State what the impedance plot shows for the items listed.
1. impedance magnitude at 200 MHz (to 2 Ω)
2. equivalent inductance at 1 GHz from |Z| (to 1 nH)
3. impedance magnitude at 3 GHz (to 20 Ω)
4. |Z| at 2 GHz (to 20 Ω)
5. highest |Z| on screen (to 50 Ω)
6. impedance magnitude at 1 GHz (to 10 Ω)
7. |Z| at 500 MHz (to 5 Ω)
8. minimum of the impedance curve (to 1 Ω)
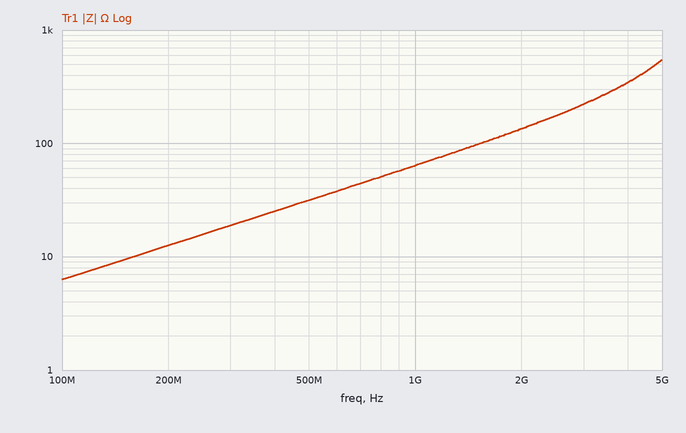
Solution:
12 Ω
10 nH
220 Ω
140 Ω
550 Ω
60 Ω
30 Ω
6 Ω
